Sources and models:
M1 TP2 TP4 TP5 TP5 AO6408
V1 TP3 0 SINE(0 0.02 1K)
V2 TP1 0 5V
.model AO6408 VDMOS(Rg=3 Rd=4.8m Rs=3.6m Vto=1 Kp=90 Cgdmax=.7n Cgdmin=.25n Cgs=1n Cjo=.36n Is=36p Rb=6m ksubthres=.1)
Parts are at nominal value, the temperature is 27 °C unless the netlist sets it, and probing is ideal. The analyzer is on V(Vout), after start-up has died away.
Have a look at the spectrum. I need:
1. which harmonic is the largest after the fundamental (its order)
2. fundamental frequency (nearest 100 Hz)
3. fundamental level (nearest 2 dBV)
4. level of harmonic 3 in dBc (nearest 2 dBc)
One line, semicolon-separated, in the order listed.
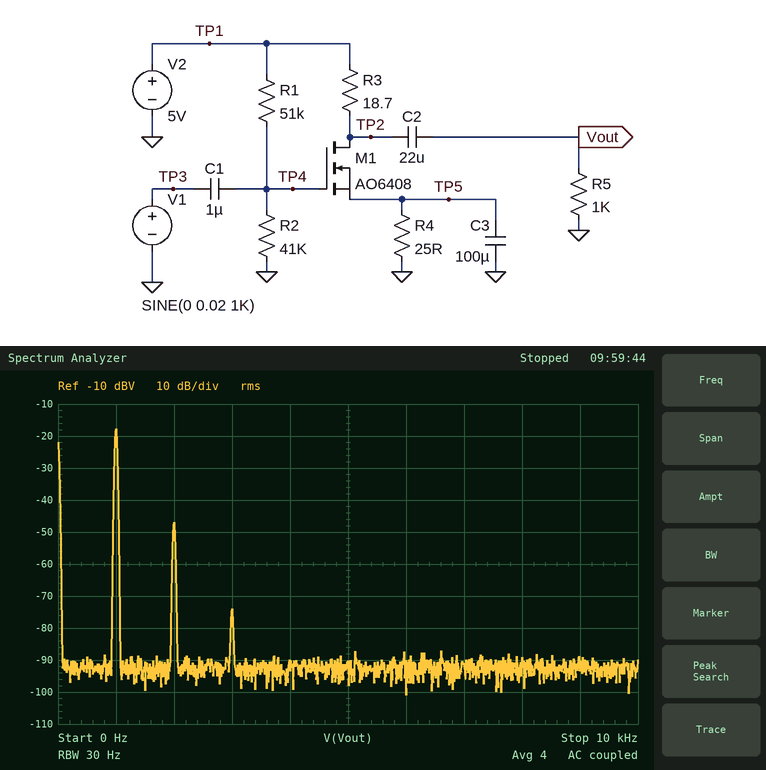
2; 1.0 kHz; -18 dBV; -56 dBc
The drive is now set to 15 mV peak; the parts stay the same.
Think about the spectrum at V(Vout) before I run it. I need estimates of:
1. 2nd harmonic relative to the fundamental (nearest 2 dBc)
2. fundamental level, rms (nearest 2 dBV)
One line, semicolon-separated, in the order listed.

-32 dBc; -20 dBV
